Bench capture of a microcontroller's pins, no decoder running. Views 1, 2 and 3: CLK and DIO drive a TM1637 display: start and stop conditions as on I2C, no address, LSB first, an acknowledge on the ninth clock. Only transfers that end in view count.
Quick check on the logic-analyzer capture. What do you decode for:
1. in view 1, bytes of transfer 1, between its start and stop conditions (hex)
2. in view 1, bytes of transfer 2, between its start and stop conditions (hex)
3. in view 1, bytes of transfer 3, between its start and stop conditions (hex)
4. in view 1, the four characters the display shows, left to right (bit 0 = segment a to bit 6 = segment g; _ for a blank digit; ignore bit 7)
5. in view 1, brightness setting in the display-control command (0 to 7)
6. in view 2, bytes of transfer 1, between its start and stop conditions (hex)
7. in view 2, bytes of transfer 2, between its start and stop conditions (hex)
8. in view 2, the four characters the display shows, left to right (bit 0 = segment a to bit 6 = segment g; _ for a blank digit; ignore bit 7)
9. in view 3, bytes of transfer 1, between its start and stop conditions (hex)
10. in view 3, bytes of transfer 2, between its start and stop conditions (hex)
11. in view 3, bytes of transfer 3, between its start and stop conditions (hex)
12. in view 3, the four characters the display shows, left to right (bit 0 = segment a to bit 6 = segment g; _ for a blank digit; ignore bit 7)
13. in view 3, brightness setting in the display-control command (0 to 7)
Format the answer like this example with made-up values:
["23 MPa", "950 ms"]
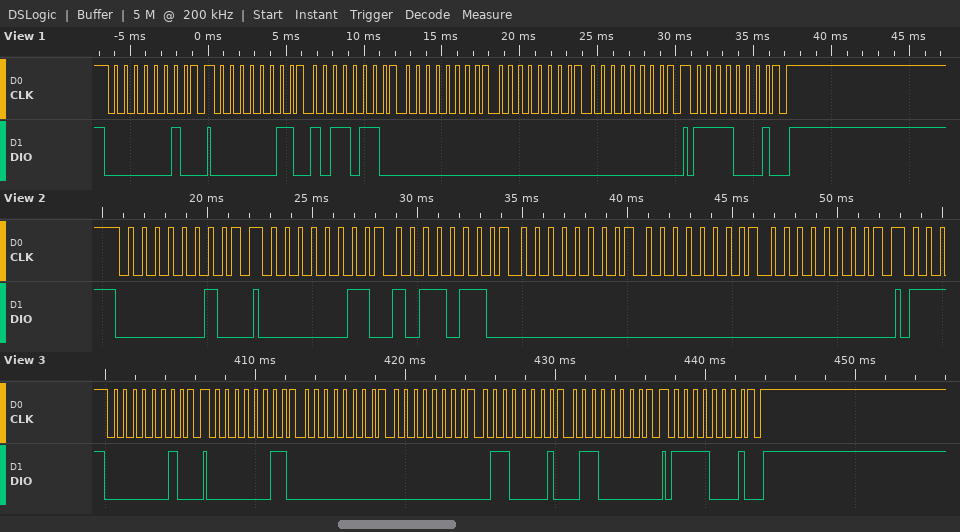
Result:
["40", "C0 6D 00 00 00", "8F", "5___", "7", "40", "C0 6D 00 00 00", "5___", "40", "C0 00 00 86 06", "8F", "__11", "7"]
